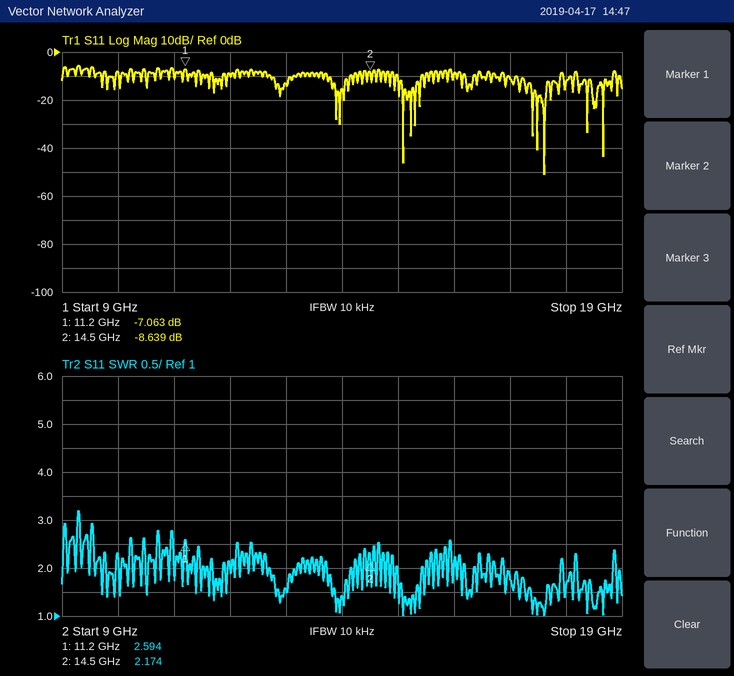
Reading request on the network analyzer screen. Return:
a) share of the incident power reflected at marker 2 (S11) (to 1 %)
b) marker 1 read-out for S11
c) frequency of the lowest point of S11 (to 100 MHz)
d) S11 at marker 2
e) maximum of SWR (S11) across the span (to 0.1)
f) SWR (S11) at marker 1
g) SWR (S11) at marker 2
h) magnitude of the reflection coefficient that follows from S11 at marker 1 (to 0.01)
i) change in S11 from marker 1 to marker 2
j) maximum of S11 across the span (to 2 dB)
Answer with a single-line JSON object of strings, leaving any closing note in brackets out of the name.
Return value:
{"share of the incident power reflected at marker 2 (S11)": "14 %", "marker 1 read-out for S11": "-7.063 dB", "frequency of the lowest point of S11": "17.6 GHz", "S11 at marker 2": "-8.639 dB", "maximum of SWR (S11) across the span": "3.2", "SWR (S11) at marker 1": "2.594", "SWR (S11) at marker 2": "2.174", "magnitude of the reflection coefficient that follows from S11 at marker 1": "0.44", "change in S11 from marker 1 to marker 2": "-1.576 dB", "maximum of S11 across the span": "-6 dB"}
